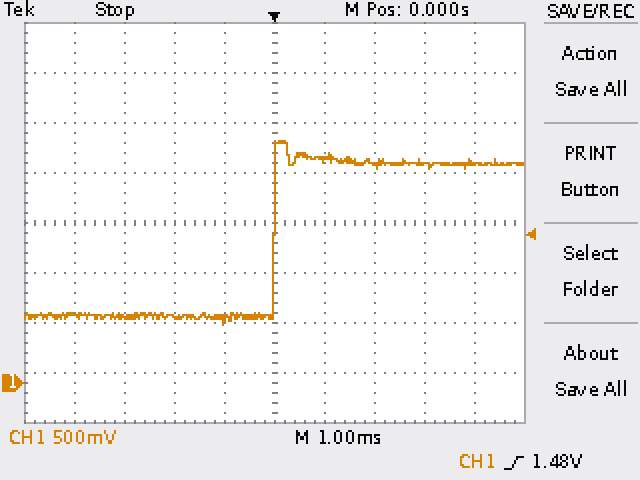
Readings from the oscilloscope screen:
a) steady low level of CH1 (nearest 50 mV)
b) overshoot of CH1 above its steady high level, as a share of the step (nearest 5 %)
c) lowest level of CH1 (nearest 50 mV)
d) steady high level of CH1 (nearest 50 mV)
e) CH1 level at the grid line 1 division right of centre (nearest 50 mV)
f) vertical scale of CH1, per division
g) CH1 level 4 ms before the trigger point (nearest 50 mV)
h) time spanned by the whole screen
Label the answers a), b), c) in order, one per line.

a) 650 mV
b) 15 %
c) 600 mV
d) 2.20 V
e) 2.25 V
f) 500 mV
g) 700 mV
h) 10 ms
